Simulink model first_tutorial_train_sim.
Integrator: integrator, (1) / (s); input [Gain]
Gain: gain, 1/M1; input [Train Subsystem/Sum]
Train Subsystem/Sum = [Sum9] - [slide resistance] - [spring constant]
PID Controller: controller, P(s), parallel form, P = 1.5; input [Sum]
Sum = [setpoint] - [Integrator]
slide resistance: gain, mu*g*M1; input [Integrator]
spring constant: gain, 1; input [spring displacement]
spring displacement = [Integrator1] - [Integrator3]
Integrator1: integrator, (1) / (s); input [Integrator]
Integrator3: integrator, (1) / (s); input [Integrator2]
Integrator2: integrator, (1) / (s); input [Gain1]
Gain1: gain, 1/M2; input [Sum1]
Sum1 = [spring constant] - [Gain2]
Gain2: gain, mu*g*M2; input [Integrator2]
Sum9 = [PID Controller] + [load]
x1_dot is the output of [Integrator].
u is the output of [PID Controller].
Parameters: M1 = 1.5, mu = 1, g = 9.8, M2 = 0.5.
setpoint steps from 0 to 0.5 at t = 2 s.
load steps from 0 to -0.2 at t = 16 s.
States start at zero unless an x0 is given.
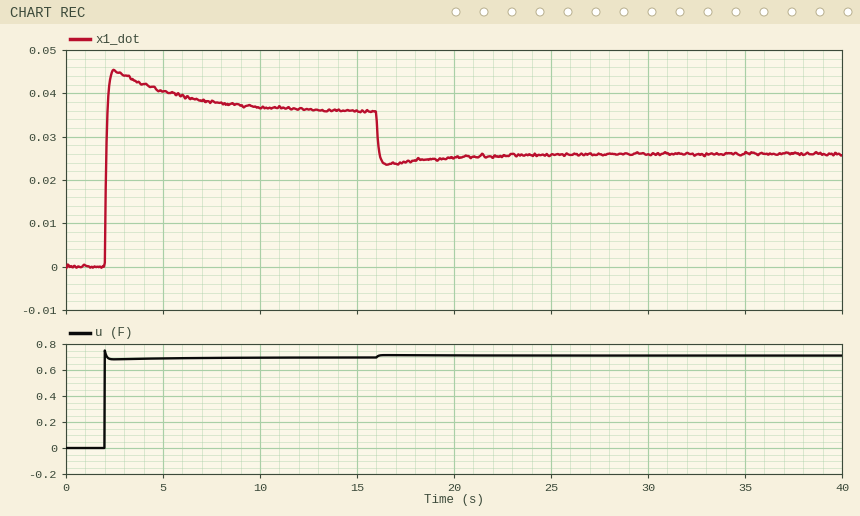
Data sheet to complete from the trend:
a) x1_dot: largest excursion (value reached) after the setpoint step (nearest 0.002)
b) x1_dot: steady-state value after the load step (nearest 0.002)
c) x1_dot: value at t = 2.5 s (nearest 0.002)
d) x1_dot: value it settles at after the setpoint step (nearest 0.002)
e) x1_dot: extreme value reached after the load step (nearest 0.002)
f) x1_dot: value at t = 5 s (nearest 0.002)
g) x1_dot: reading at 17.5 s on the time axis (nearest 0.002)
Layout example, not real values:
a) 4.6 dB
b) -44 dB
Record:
a) 0.046
b) 0.026
c) 0.046
d) 0.036
e) 0.024
f) 0.040
g) 0.024
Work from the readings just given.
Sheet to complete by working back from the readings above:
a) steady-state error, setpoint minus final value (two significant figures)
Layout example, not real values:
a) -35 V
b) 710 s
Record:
a) 0.46
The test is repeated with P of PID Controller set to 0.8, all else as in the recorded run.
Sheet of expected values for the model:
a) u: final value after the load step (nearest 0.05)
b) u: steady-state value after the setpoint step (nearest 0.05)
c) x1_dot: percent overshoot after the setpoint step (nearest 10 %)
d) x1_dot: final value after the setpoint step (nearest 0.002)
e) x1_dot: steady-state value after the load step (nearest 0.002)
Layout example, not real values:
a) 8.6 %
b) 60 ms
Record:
a) 0.40
b) 0.40
c) 30 %
d) 0.020
e) 0.010
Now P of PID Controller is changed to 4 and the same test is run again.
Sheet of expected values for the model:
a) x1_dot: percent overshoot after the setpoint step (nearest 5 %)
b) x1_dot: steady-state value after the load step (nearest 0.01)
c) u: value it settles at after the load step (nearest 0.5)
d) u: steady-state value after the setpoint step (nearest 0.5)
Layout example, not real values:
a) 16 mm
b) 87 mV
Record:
a) 25 %
b) 0.08
c) 1.5
d) 1.5
